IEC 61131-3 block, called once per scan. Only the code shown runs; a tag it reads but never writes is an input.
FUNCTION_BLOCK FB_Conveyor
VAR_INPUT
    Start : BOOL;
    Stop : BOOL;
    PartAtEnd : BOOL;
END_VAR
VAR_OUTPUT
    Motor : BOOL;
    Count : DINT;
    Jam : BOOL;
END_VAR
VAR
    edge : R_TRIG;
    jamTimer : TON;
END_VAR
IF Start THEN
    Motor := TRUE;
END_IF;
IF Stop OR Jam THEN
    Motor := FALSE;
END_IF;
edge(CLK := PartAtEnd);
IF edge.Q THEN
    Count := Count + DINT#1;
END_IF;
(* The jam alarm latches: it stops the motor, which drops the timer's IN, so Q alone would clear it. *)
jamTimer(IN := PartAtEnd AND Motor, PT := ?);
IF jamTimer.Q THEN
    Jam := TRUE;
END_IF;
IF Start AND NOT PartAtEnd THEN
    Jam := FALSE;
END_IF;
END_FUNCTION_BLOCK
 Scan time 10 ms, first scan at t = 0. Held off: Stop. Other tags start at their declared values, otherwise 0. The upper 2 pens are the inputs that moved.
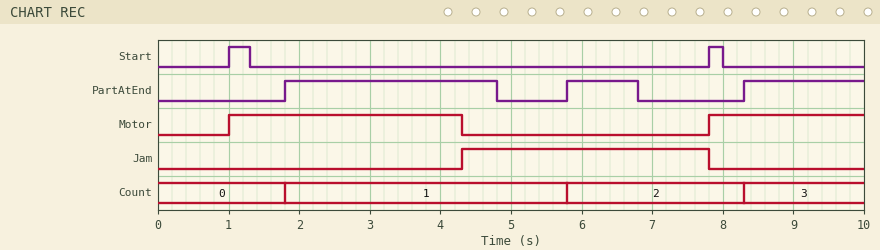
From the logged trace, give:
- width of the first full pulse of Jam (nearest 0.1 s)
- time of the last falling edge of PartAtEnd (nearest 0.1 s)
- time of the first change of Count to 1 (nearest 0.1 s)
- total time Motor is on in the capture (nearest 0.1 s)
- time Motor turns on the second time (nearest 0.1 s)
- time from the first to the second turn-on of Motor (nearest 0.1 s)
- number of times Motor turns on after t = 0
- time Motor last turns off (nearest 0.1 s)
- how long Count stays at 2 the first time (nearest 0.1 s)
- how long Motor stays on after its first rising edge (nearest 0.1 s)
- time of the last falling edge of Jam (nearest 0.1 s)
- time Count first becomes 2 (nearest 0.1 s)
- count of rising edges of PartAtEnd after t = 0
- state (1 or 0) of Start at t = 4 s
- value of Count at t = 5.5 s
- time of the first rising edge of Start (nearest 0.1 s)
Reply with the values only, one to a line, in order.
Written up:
3.5 s
6.8 s
1.8 s
5.5 s
7.8 s
6.8 s
2
4.3 s
2.5 s
3.3 s
7.8 s
5.8 s
3
0
1
1.0 s
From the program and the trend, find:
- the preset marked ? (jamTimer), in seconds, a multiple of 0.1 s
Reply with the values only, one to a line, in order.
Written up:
2.5 s
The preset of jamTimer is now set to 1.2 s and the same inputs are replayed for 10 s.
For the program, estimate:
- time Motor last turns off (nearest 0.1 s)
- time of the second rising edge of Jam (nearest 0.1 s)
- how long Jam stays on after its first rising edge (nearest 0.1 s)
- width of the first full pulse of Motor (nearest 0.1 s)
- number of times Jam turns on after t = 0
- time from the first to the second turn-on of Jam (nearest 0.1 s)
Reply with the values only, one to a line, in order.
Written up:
9.5 s
9.5 s
4.8 s
2.0 s
2
6.5 s
